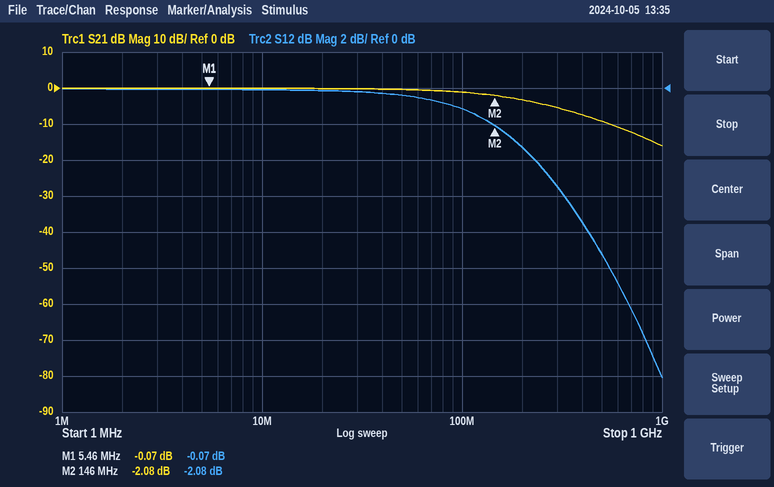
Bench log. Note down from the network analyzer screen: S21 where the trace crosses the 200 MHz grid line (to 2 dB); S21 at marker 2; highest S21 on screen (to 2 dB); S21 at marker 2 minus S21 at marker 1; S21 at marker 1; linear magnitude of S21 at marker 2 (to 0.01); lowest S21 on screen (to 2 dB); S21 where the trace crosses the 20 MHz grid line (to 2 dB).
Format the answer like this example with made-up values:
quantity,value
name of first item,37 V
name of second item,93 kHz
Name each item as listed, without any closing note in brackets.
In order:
quantity,value
S21 where the trace crosses the 200 MHz grid line,-4 dB
S21 at marker 2,-2.08 dB
highest S21 on screen,0 dB
S21 at marker 2 minus S21 at marker 1,-2.01 dB
S21 at marker 1,-0.07 dB
linear magnitude of S21 at marker 2,0.79
lowest S21 on screen,-16 dB
S21 where the trace crosses the 20 MHz grid line,0 dB
